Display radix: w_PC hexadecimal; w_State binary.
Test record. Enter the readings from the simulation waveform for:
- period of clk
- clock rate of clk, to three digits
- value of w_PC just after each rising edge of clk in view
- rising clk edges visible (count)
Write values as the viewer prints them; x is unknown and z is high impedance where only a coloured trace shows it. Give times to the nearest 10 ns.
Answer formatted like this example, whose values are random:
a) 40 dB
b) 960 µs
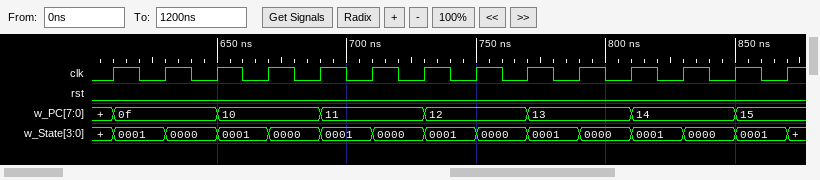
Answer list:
a) 20 ns
b) 50.0 MHz
c) 0f, 0f, 10, 10, 11, 11, 12, 12, 13, 13, 14, 14, 15, 15
d) 14
